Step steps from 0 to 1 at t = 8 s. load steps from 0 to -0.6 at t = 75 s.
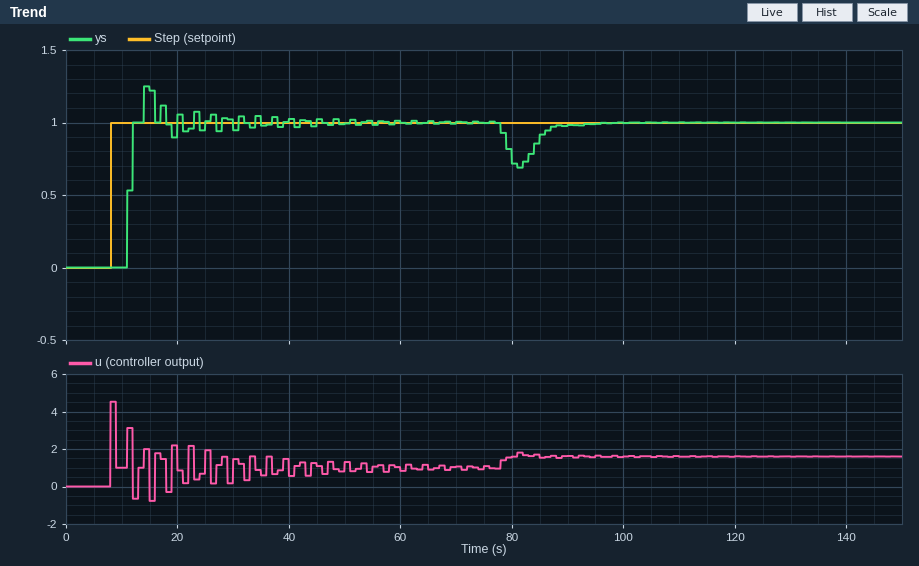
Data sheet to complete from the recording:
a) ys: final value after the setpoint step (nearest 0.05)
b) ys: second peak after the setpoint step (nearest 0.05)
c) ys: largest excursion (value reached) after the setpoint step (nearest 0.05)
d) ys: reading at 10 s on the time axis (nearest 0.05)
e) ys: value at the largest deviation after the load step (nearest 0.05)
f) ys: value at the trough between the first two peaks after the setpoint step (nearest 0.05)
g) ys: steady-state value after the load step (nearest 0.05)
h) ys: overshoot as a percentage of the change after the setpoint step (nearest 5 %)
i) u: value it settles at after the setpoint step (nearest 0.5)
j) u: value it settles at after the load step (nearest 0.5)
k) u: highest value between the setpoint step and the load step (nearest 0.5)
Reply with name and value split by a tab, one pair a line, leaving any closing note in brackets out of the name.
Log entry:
ys: final value after the setpoint step	1.00
ys: second peak after the setpoint step	1.10
ys: largest excursion (value reached) after the setpoint step	1.25
ys: reading at 10 s on the time axis	0.00
ys: value at the largest deviation after the load step	0.70
ys: value at the trough between the first two peaks after the setpoint step	1.00
ys: steady-state value after the load step	1.00
ys: overshoot as a percentage of the change after the setpoint step	25 %
u: value it settles at after the setpoint step	1.0
u: value it settles at after the load step	1.5
u: highest value between the setpoint step and the load step	4.5
